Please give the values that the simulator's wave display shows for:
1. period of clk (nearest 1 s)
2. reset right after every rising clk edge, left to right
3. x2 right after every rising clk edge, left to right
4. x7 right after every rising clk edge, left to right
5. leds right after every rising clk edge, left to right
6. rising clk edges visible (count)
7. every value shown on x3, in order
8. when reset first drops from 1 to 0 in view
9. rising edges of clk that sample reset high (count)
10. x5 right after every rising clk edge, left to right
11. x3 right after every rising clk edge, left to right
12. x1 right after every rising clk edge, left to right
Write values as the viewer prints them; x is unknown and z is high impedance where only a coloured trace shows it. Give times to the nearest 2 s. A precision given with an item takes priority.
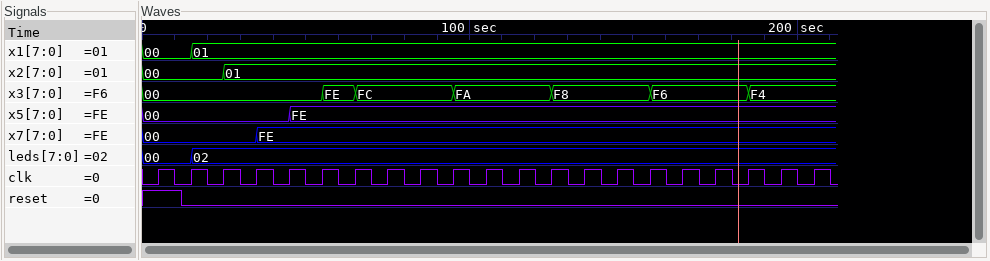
10 s
1 0 0 0 0 0 0 0 0 0 0 0 0 0 0 0 0 0 0 0 0
00, 00, 01, 01, 01, 01, 01, 01, 01, 01, 01, 01, 01, 01, 01, 01, 01, 01, 01, 01, 01
00, 00, 00, FE, FE, FE, FE, FE, FE, FE, FE, FE, FE, FE, FE, FE, FE, FE, FE, FE, FE
00, 02, 02, 02, 02, 02, 02, 02, 02, 02, 02, 02, 02, 02, 02, 02, 02, 02, 02, 02, 02
21
00, FE, FC, FA, F8, F6, F4
12 s
1
00, 00, 00, 00, FE, FE, FE, FE, FE, FE, FE, FE, FE, FE, FE, FE, FE, FE, FE, FE, FE
00, 00, 00, 00, 00, FE, FC, FC, FC, FA, FA, FA, F8, F8, F8, F6, F6, F6, F4, F4, F4
00, 01, 01, 01, 01, 01, 01, 01, 01, 01, 01, 01, 01, 01, 01, 01, 01, 01, 01, 01, 01
